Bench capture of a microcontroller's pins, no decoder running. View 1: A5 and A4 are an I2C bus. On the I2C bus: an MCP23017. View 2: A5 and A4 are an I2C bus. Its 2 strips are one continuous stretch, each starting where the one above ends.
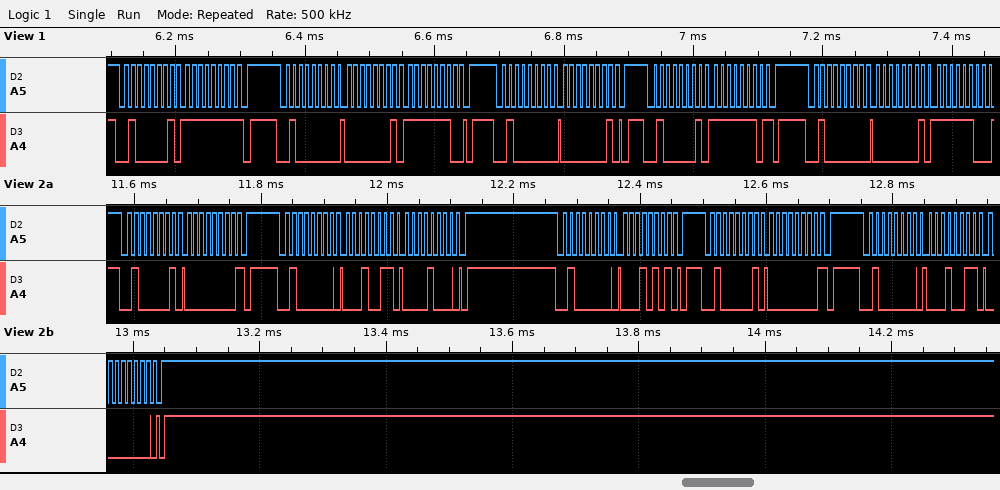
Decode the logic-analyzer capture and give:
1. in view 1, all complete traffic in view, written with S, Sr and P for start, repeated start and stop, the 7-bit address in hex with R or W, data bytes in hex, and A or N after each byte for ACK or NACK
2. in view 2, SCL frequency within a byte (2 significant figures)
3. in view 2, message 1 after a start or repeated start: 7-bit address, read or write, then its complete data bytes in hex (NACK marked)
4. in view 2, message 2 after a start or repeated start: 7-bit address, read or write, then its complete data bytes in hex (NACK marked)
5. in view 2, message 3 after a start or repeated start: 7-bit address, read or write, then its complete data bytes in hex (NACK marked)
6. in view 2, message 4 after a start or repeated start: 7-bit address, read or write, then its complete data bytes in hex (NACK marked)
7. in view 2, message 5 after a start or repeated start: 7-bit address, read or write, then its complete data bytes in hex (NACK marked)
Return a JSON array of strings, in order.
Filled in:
["S 20R A FF N P S 20W A 01 A FE A P S 20W A 01 A P S 20R A FE N P S 20W A 01 A FC A", "100 kHz", "0x20 read: 00 NACK", "0x20 write: 13 08", "0x20 write: 15", "0x20 read: 00 NACK", "0x20 write: 13 00"]
